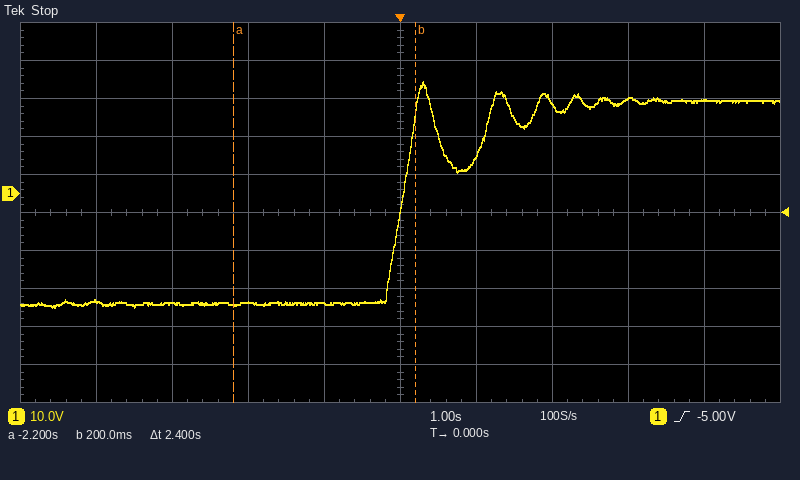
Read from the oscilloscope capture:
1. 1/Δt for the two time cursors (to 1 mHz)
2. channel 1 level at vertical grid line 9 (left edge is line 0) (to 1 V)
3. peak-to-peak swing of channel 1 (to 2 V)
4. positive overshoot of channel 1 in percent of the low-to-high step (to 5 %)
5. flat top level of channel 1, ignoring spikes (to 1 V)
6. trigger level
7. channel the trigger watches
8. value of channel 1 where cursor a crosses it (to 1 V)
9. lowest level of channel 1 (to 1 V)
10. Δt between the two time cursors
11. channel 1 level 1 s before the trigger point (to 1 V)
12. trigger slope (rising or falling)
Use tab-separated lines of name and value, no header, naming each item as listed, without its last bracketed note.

1/Δt for the two time cursors	417 mHz
channel 1 level at vertical grid line 9 (left edge is line 0)	25 V
peak-to-peak swing of channel 1	60 V
positive overshoot of channel 1 in percent of the low-to-high step	10 %
flat top level of channel 1, ignoring spikes	24 V
trigger level	-5.00 V
channel the trigger watches	channel 1
value of channel 1 where cursor a crosses it	-29 V
lowest level of channel 1	-30 V
Δt between the two time cursors	2.4 s
channel 1 level 1 s before the trigger point	-29 V
trigger slope	rising
